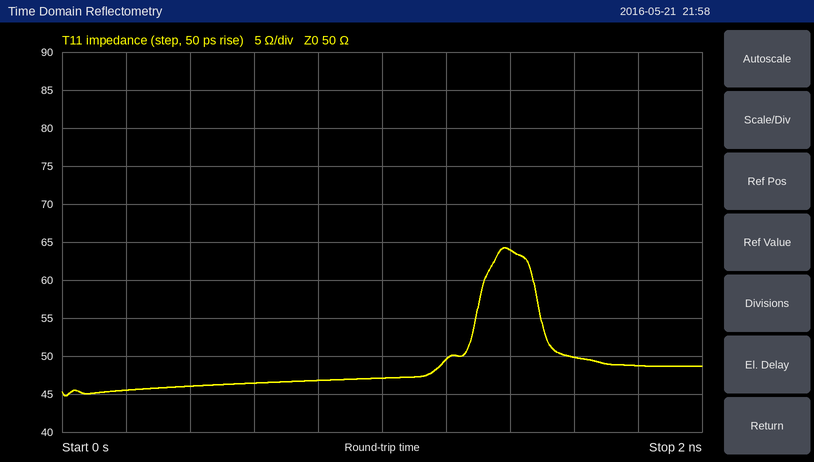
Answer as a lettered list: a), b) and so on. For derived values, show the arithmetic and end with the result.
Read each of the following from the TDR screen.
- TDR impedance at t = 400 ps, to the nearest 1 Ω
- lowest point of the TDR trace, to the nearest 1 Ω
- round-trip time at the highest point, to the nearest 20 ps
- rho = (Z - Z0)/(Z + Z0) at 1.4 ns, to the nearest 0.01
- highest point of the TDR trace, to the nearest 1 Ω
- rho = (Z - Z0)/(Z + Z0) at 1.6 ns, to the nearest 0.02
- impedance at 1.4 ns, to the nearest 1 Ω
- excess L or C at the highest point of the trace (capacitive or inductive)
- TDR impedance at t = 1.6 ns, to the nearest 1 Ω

a) 46 Ω
b) 45 Ω
c) 1.38 ns
d) (64 − 50)/(64 + 50) ≈ +0.12
e) 64 Ω
f) (50 − 50)/(50 + 50) ≈ 0.00
g) 64 Ω
h) inductive
i) 50 Ω
